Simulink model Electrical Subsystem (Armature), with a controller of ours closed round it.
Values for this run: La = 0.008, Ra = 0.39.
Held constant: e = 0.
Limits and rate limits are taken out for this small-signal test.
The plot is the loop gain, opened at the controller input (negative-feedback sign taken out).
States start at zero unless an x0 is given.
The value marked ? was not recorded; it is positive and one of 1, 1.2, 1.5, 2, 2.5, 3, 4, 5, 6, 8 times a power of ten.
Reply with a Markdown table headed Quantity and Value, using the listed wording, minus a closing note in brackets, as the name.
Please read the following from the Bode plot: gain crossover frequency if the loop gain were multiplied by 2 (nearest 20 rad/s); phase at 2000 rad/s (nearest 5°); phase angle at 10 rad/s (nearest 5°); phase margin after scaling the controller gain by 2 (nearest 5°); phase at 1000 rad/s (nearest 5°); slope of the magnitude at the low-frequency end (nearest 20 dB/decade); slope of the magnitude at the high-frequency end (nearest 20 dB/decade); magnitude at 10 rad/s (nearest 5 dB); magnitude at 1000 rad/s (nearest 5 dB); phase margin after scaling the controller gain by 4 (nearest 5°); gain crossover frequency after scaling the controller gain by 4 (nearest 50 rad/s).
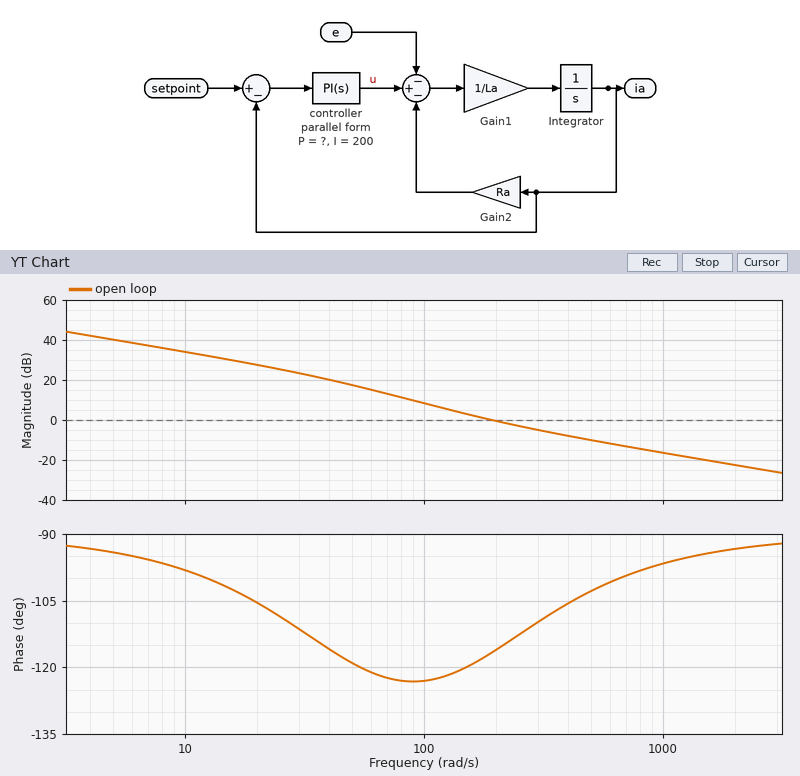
| Quantity | Value |
|---|---|
| gain crossover frequency if the loop gain were multiplied by 2 | 340 rad/s |
| phase at 2000 rad/s | -95° |
| phase angle at 10 rad/s | -100° |
| phase margin after scaling the controller gain by 2 | 70° |
| phase at 1000 rad/s | -95° |
| slope of the magnitude at the low-frequency end | -20 dB/decade |
| slope of the magnitude at the high-frequency end | -20 dB/decade |
| magnitude at 10 rad/s | 35 dB |
| magnitude at 1000 rad/s | -15 dB |
| phase margin after scaling the controller gain by 4 | 80° |
| gain crossover frequency after scaling the controller gain by 4 | 600 rad/s |
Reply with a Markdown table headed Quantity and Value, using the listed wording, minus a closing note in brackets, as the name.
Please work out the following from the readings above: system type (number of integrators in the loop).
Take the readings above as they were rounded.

| Quantity | Value |
|---|---|
| system type | 1 |
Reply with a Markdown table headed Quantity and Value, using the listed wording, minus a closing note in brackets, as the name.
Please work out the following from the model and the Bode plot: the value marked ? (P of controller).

| Quantity | Value |
|---|---|
| the value marked ? | 1.2 |
